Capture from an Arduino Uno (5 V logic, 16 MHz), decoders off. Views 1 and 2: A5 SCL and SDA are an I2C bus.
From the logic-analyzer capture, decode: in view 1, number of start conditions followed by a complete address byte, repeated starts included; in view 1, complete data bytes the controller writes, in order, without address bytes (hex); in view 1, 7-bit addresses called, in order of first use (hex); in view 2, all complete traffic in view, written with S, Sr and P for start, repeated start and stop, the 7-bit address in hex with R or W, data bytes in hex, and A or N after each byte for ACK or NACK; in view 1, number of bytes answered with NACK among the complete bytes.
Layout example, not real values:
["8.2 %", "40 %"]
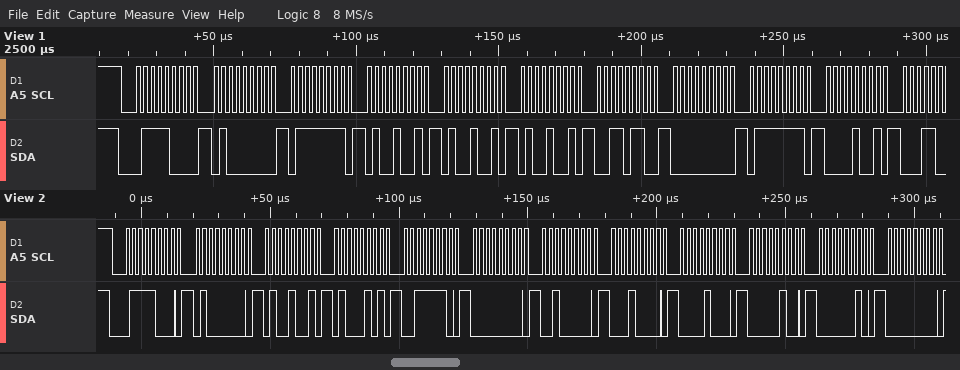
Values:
["1", "40 7F 49 49 49 36 00 7F 09", "0x3C", "S 3CW A 40 A 49 A 45 A 3E A 00 A 20 A 10 A 08 A 04 A 02 A 00 A", "0"]
